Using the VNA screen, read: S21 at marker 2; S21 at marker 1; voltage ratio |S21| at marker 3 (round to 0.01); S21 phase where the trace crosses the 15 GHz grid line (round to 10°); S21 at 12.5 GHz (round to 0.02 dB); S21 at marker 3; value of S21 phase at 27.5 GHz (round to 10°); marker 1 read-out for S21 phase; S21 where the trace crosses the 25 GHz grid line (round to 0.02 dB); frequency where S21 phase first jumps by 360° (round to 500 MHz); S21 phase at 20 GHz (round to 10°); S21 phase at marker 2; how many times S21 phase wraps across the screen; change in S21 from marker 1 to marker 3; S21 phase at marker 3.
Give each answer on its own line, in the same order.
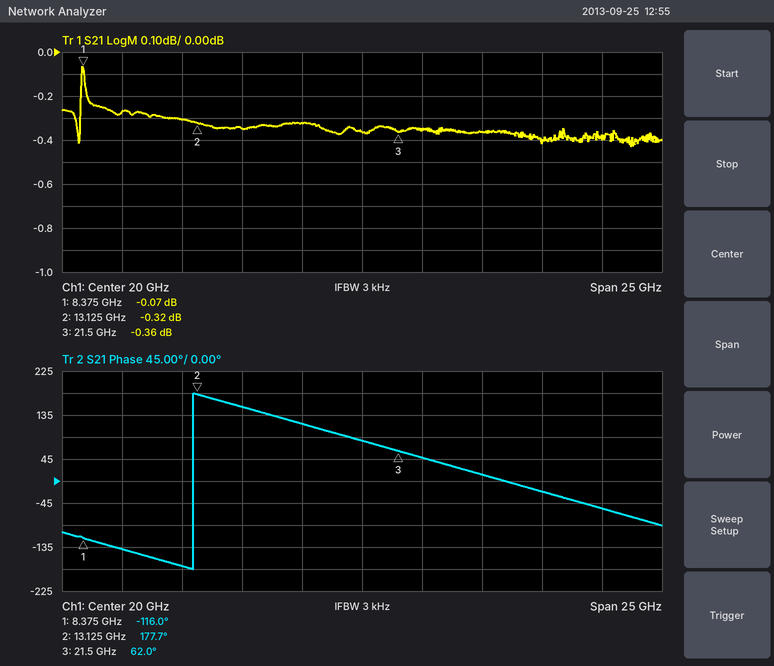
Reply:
-0.32 dB
-0.07 dB
0.96
150°
-0.30 dB
-0.36 dB
-20°
-116.0°
-0.36 dB
13.0 GHz
80°
177.7°
1
-0.29 dB
62.0°
